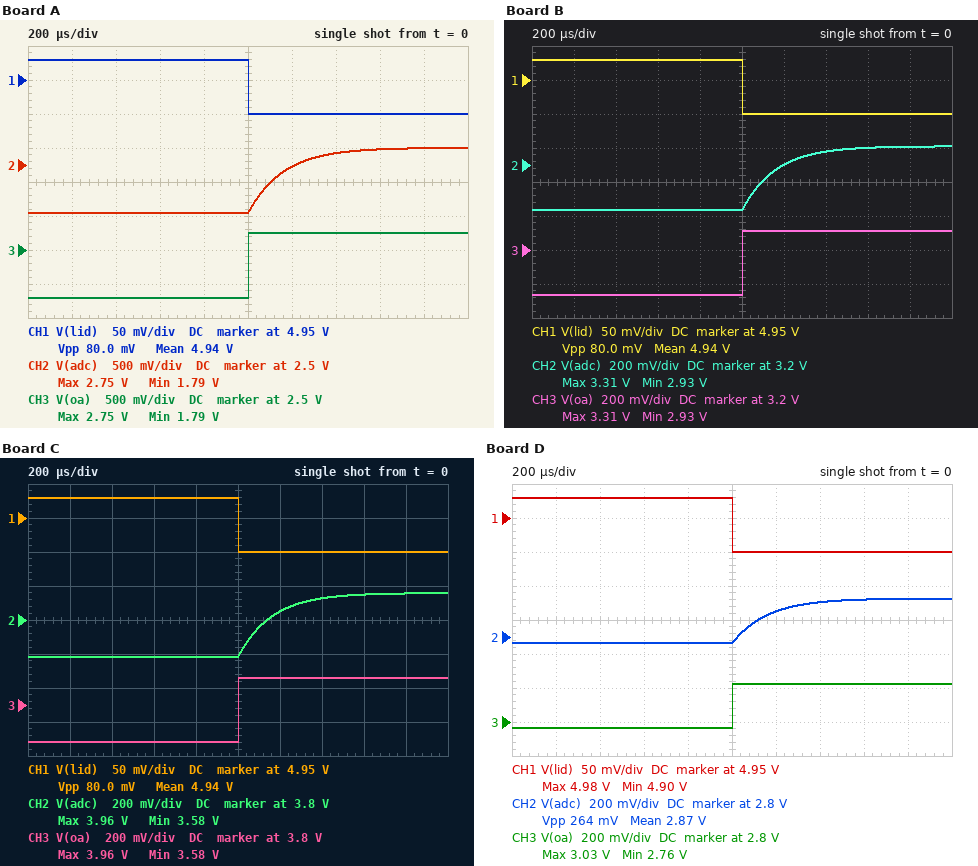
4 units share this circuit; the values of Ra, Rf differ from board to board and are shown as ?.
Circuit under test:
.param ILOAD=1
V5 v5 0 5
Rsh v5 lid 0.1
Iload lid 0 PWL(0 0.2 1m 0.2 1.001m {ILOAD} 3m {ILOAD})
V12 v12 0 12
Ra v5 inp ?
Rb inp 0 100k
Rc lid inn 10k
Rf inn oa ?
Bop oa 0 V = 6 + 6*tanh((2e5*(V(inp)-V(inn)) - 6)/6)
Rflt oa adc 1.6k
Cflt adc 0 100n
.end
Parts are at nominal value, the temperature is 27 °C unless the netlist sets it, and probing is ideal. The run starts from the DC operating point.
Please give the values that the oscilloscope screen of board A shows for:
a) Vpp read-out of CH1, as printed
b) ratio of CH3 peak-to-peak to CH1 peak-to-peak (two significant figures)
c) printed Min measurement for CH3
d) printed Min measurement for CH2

80.0 mV
12
1.79 V
1.79 V
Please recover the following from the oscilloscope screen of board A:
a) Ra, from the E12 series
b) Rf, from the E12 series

5.6 kΩ
120 kΩ
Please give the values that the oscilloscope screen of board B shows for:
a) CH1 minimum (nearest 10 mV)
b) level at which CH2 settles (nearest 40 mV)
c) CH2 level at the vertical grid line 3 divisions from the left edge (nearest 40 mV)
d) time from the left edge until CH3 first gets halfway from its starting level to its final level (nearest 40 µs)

4.90 V
3.32 V
2.92 V
1.00 ms
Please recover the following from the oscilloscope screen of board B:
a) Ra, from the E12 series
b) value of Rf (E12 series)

8.2 kΩ
47 kΩ
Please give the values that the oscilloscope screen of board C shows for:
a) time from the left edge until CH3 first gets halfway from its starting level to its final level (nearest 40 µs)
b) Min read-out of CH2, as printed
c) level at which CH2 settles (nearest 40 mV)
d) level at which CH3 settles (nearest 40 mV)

1.00 ms
3.58 V
3.96 V
3.96 V
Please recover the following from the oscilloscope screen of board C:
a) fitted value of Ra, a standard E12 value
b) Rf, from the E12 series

5.6 kΩ
47 kΩ
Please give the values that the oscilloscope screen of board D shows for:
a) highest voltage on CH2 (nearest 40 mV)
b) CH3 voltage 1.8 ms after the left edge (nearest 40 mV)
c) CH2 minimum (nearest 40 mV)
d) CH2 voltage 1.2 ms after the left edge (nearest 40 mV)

3.04 V
3.04 V
2.76 V
2.96 V
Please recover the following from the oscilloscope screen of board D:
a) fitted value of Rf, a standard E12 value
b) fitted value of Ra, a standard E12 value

33 kΩ
12 kΩ
